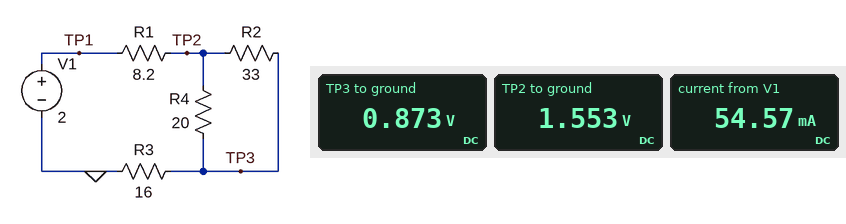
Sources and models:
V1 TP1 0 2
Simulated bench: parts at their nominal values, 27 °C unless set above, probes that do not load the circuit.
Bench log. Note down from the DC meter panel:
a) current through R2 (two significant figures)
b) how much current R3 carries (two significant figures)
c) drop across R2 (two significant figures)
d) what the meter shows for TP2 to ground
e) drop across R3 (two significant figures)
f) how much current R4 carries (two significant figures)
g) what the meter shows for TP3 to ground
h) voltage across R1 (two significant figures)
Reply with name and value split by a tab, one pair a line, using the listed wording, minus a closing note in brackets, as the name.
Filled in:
current through R2	21 mA
how much current R3 carries	55 mA
drop across R2	680 mV
what the meter shows for TP2 to ground	1.553 V
drop across R3	870 mV
how much current R4 carries	34 mA
what the meter shows for TP3 to ground	0.873 V
voltage across R1	450 mV
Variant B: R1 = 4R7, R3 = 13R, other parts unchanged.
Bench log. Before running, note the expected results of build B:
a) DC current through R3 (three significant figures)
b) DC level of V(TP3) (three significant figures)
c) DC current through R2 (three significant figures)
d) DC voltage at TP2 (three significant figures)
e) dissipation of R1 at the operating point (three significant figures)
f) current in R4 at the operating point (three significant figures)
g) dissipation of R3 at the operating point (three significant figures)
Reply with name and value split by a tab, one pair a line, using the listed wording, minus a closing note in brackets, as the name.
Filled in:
DC current through R3	66.3 mA
DC level of V(TP3)	862 mV
DC current through R2	25.0 mA
DC voltage at TP2	1.69 V
dissipation of R1 at the operating point	20.7 mW
current in R4 at the operating point	41.3 mA
dissipation of R3 at the operating point	57.2 mW
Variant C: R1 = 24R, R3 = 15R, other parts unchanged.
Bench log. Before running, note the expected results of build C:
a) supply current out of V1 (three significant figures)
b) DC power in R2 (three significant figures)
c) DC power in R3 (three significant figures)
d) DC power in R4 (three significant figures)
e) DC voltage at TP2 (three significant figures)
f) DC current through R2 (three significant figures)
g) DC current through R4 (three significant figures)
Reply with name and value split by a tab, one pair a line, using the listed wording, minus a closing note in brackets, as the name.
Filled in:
supply current out of V1	38.9 mA
DC power in R2	7.10 mW
DC power in R3	22.7 mW
DC power in R4	11.7 mW
DC voltage at TP2	1.07 V
DC current through R2	14.7 mA
DC current through R4	24.2 mA
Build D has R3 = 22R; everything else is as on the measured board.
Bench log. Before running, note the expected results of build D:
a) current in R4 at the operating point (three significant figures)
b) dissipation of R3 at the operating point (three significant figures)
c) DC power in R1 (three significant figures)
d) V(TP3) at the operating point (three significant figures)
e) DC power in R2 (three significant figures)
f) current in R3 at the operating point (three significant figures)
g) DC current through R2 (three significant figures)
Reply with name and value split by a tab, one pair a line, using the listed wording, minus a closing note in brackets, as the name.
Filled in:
current in R4 at the operating point	29.2 mA
dissipation of R3 at the operating point	48.4 mW
DC power in R1	18.0 mW
V(TP3) at the operating point	1.03 V
DC power in R2	10.3 mW
current in R3 at the operating point	46.9 mA
DC current through R2	17.7 mA
